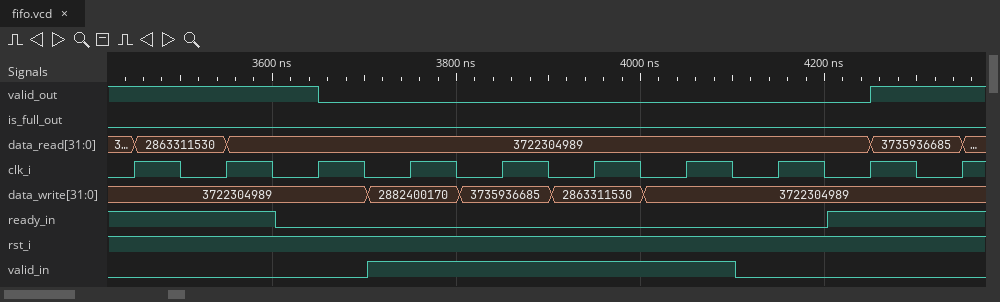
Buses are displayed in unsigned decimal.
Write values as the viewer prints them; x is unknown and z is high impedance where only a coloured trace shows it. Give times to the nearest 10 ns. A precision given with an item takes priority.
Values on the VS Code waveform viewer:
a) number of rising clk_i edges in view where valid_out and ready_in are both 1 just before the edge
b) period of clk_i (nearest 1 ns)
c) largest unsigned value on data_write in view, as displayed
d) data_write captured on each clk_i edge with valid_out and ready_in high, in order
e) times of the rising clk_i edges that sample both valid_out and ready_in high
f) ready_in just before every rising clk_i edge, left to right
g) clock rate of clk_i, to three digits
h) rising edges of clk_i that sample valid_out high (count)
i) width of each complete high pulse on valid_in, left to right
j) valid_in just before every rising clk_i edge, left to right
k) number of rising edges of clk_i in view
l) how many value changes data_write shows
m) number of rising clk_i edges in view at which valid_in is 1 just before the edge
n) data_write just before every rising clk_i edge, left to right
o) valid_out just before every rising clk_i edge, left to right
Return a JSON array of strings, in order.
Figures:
["3", "100 ns", "3735936685", "3722304989, 3722304989, 3722304989", "3450 ns, 3550 ns, 4350 ns", "1 1 0 0 0 0 0 0 1 1", "10.0 MHz", "4", "400 ns", "0 0 0 1 1 1 1 0 0 0", "10", "4", "4", "3722304989, 3722304989, 3722304989, 2882400170, 3735936685, 2863311530, 3722304989, 3722304989, 3722304989, 3722304989", "1 1 1 0 0 0 0 0 0 1"]
